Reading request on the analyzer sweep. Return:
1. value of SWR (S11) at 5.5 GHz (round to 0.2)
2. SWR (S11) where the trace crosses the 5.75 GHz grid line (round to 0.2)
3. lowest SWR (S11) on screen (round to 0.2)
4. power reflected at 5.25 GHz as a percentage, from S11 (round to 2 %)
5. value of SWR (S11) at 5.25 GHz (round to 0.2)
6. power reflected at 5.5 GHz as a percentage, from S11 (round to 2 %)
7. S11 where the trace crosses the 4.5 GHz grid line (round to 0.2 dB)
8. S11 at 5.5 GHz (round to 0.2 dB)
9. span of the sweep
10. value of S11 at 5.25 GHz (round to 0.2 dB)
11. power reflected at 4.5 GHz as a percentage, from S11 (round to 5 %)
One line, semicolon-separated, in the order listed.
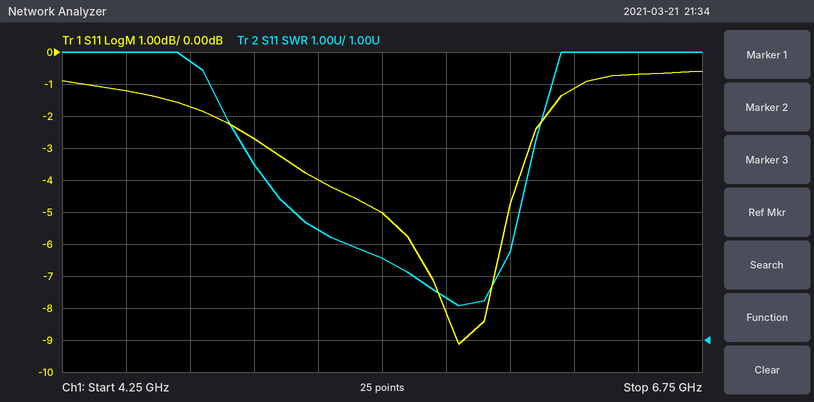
3.6; 2.4; 2.0; 40 %; 4.4; 32 %; -1.2 dB; -5.0 dB; 2.5 GHz; -4.0 dB; 75 %
